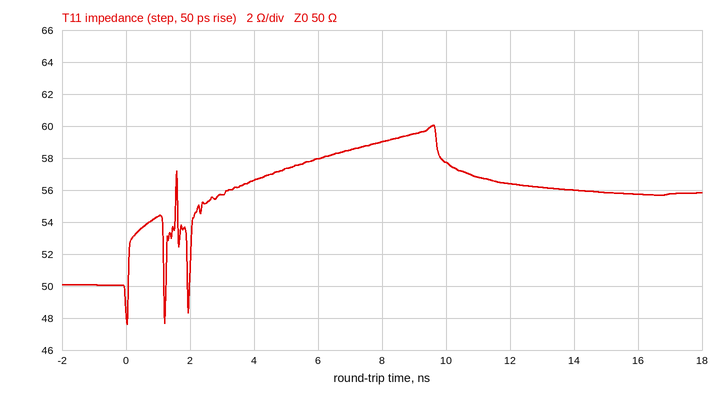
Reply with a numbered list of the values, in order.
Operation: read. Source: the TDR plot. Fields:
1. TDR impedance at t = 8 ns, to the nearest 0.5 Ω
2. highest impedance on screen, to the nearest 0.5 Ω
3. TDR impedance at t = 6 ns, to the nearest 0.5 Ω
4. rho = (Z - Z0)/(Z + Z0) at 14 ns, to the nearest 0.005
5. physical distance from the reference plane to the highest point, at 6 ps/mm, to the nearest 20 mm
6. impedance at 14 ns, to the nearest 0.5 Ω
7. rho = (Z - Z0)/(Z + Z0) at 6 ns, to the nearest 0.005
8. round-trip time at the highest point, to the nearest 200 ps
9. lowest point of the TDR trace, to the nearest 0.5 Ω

1. 59.0 Ω
2. 60.0 Ω
3. 58.0 Ω
4. +0.055
5. 800 mm
6. 56.0 Ω
7. +0.075
8. 9.6 ns
9. 47.5 Ω
